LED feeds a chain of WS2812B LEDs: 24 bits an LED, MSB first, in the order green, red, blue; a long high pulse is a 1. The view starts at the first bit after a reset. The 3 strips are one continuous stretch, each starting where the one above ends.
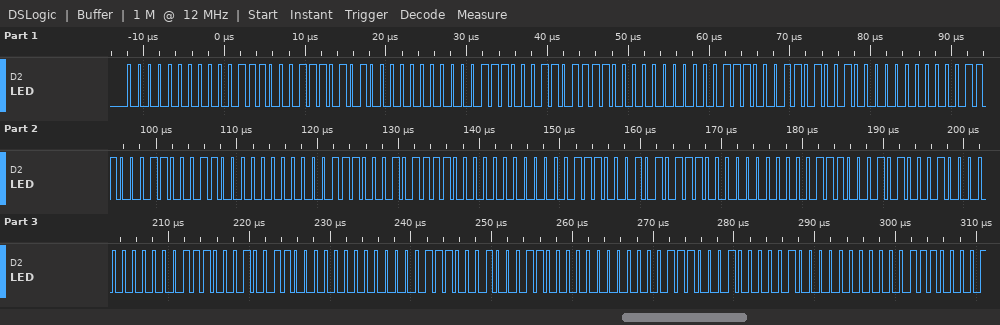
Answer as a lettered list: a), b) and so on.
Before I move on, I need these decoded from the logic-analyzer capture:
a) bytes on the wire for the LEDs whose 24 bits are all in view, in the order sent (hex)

a) 00 1C 75 00 1C 6F 00 1C 69 00 1C 63 00 1C 5E 00 1C 57 00 1C 51 00 1C 4C 00 1C 46 00 1C 41
